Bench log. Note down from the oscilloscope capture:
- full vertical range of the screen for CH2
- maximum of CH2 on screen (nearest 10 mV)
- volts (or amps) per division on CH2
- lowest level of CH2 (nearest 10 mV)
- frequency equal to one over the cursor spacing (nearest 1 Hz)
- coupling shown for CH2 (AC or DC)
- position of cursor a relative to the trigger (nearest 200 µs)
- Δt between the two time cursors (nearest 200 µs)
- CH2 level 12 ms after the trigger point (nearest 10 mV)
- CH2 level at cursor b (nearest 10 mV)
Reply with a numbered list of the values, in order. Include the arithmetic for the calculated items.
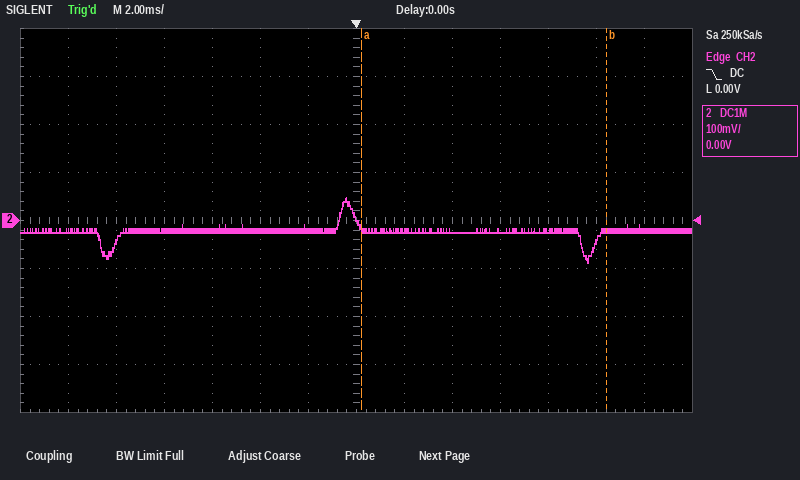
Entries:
1. 800 mV
2. 50 mV
3. 100 mV
4. -90 mV
5. 1 / 10.2 ms ≈ 98 Hz
6. DC
7. +200 µs
8. 10.2 ms
9. -20 mV
10. -20 mV
